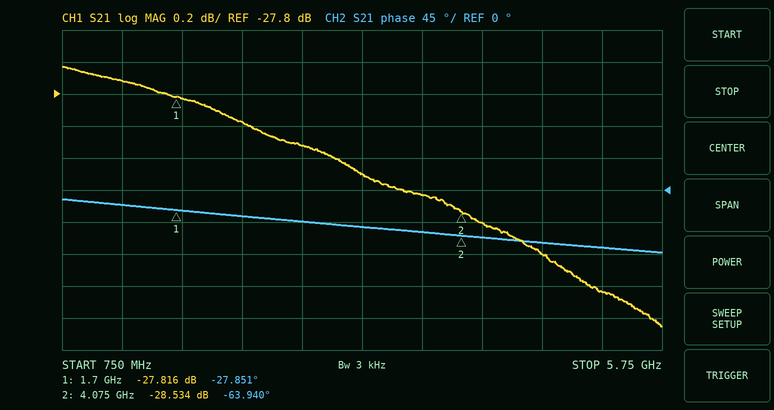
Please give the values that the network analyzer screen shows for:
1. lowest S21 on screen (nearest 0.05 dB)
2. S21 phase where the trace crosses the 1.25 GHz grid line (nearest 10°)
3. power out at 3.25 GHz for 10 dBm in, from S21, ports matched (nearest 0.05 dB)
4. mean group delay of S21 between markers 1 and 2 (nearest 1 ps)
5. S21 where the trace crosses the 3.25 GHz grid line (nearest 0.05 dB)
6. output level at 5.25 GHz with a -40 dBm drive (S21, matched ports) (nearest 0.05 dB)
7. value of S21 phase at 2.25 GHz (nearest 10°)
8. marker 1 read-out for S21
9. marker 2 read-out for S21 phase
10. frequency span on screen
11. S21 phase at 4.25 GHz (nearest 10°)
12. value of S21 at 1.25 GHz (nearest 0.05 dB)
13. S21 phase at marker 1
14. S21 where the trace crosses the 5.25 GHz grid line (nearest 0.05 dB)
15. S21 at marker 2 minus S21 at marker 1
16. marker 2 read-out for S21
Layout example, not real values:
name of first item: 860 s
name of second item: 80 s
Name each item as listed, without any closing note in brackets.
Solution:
lowest S21 on screen: -29.25 dB
S21 phase where the trace crosses the 1.25 GHz grid line: -20°
power out at 3.25 GHz for 10 dBm in, from S21, ports matched: -18.30 dBm
mean group delay of S21 between markers 1 and 2: 42 ps
S21 where the trace crosses the 3.25 GHz grid line: -28.30 dB
output level at 5.25 GHz with a -40 dBm drive (S21, matched ports): -69.05 dBm
value of S21 phase at 2.25 GHz: -40°
marker 1 read-out for S21: -27.816 dB
marker 2 read-out for S21 phase: -63.940°
frequency span on screen: 5 GHz
S21 phase at 4.25 GHz: -70°
value of S21 at 1.25 GHz: -27.70 dB
S21 phase at marker 1: -27.851°
S21 where the trace crosses the 5.25 GHz grid line: -29.05 dB
S21 at marker 2 minus S21 at marker 1: -0.718 dB
marker 2 read-out for S21: -28.534 dB
